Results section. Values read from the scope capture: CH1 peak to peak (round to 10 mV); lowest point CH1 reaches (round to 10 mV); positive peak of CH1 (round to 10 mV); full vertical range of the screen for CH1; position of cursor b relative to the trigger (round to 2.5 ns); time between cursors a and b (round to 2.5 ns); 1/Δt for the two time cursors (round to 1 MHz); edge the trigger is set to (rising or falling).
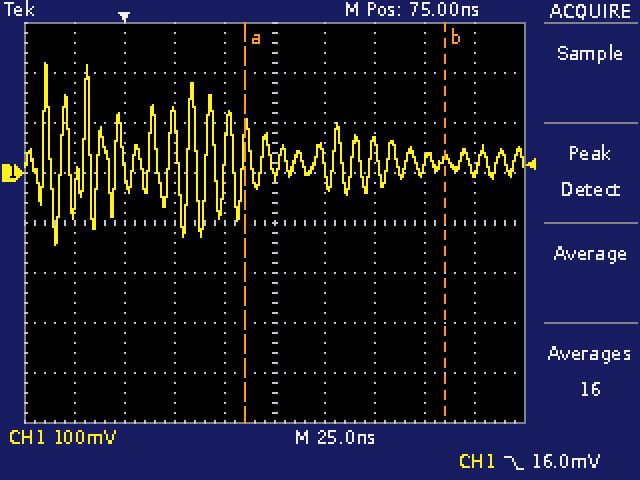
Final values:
360 mV
-140 mV
220 mV
800 mV
+160.0 ns
100.0 ns
10 MHz
falling
